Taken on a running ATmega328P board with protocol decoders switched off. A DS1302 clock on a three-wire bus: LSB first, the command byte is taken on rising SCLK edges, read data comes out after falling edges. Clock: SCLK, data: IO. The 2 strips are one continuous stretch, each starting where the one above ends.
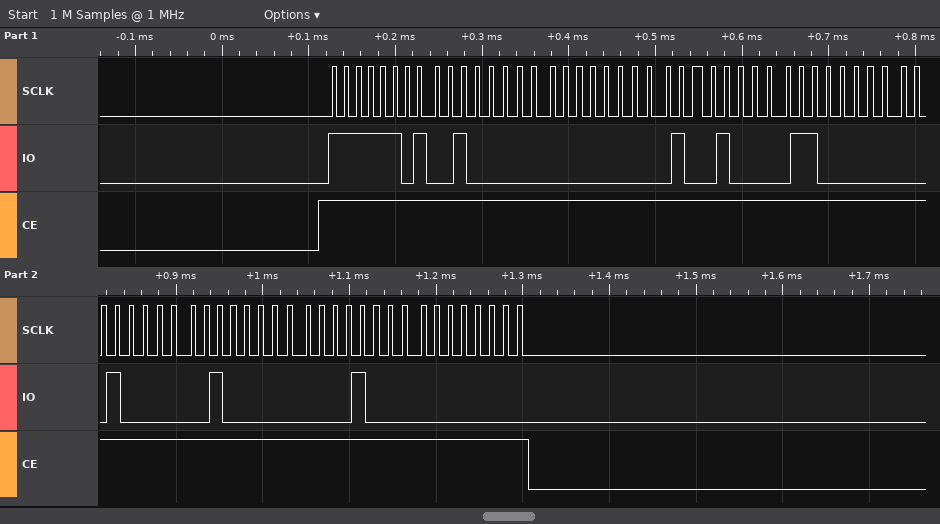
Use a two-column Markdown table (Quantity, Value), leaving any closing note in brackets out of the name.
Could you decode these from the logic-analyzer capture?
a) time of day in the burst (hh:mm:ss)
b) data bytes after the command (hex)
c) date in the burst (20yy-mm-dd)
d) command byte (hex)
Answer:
| Quantity | Value |
|---|---|
| time of day in the burst | 12:00:04 |
| data bytes after the command | 04 00 12 06 08 04 10 00 |
| date in the burst | 2010-08-06 |
| command byte | 0xBF |
